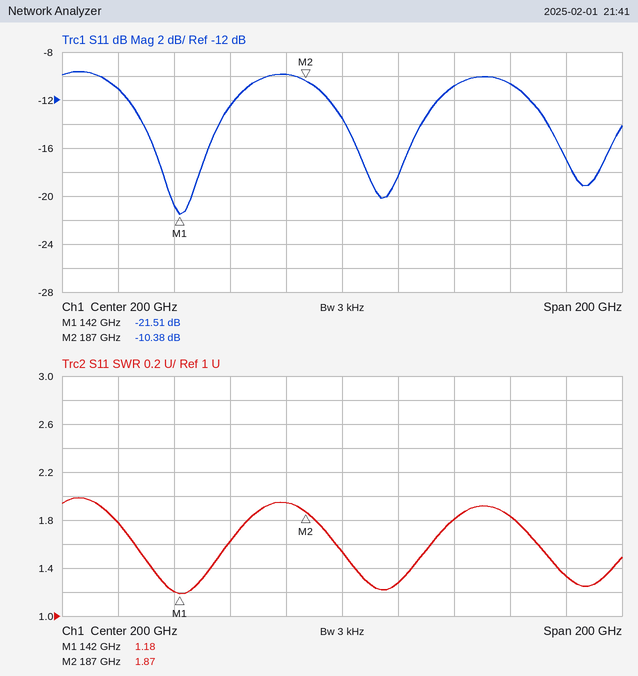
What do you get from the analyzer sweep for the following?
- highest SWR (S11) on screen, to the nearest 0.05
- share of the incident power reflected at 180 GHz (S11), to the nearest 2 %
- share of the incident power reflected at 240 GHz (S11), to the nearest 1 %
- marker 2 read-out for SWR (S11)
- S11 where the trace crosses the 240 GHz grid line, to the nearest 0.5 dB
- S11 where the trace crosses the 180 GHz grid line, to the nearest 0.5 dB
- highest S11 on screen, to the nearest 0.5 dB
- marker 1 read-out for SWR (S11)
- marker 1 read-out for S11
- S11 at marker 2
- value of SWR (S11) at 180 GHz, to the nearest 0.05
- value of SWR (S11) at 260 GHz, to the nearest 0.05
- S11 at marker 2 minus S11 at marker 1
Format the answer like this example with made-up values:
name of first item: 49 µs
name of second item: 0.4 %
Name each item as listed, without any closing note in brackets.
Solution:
highest SWR (S11) on screen, to the nearest 0.05: 2.00
share of the incident power reflected at 180 GHz (S11), to the nearest 2 %: 10 %
share of the incident power reflected at 240 GHz (S11), to the nearest 1 %: 8 %
marker 2 read-out for SWR: 1.87
S11 where the trace crosses the 240 GHz grid line, to the nearest 0.5 dB: -11.0 dB
S11 where the trace crosses the 180 GHz grid line, to the nearest 0.5 dB: -10.0 dB
highest S11 on screen, to the nearest 0.5 dB: -9.5 dB
marker 1 read-out for SWR: 1.18
marker 1 read-out for S11: -21.51 dB
S11 at marker 2: -10.38 dB
value of SWR (S11) at 180 GHz, to the nearest 0.05: 1.95
value of SWR (S11) at 260 GHz, to the nearest 0.05: 1.85
S11 at marker 2 minus S11 at marker 1: 11.13 dB
